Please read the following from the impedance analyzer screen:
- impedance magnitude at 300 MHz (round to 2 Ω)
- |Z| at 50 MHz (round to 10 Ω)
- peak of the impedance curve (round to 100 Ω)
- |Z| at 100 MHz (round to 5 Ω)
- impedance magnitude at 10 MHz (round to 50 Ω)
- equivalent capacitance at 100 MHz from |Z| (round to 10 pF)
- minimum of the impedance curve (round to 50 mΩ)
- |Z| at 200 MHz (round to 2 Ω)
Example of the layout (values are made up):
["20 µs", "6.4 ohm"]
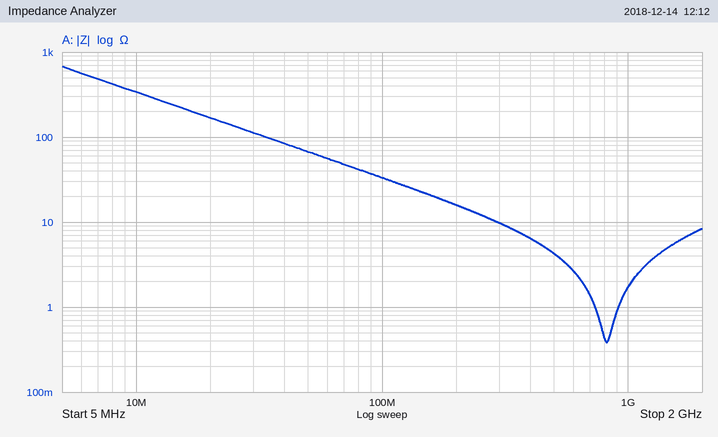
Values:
["10 Ω", "70 Ω", "700 Ω", "35 Ω", "350 Ω", "50 pF", "400 mΩ", "16 Ω"]
